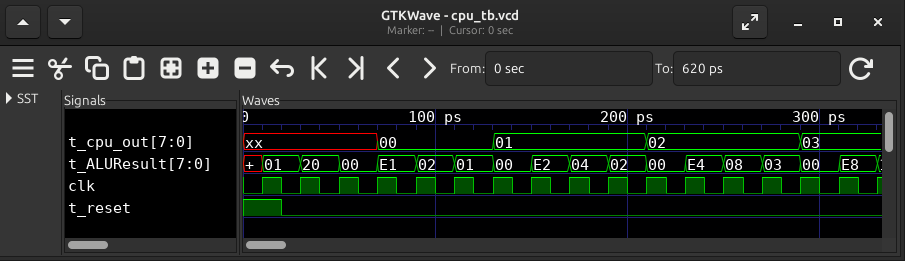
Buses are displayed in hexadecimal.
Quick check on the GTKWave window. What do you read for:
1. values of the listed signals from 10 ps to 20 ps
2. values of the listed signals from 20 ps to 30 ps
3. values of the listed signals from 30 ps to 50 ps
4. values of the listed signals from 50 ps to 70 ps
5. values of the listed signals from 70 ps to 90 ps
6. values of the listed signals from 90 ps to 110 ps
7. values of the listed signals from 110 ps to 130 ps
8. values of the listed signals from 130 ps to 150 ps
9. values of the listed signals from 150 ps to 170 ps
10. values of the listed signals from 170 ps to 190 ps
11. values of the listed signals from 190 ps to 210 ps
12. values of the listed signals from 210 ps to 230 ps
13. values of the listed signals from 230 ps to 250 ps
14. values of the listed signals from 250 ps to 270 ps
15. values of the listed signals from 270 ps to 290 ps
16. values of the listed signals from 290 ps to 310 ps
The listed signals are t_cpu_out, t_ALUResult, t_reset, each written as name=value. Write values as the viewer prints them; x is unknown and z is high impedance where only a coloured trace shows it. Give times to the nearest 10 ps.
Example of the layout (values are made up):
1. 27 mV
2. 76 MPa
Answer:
1. t_cpu_out=xx, t_ALUResult=01, t_reset=1
2. t_cpu_out=xx, t_ALUResult=01, t_reset=0
3. t_cpu_out=xx, t_ALUResult=20, t_reset=0
4. t_cpu_out=xx, t_ALUResult=00, t_reset=0
5. t_cpu_out=00, t_ALUResult=E1, t_reset=0
6. t_cpu_out=00, t_ALUResult=02, t_reset=0
7. t_cpu_out=00, t_ALUResult=01, t_reset=0
8. t_cpu_out=01, t_ALUResult=00, t_reset=0
9. t_cpu_out=01, t_ALUResult=E2, t_reset=0
10. t_cpu_out=01, t_ALUResult=04, t_reset=0
11. t_cpu_out=01, t_ALUResult=02, t_reset=0
12. t_cpu_out=02, t_ALUResult=00, t_reset=0
13. t_cpu_out=02, t_ALUResult=E4, t_reset=0
14. t_cpu_out=02, t_ALUResult=08, t_reset=0
15. t_cpu_out=02, t_ALUResult=03, t_reset=0
16. t_cpu_out=03, t_ALUResult=00, t_reset=0
